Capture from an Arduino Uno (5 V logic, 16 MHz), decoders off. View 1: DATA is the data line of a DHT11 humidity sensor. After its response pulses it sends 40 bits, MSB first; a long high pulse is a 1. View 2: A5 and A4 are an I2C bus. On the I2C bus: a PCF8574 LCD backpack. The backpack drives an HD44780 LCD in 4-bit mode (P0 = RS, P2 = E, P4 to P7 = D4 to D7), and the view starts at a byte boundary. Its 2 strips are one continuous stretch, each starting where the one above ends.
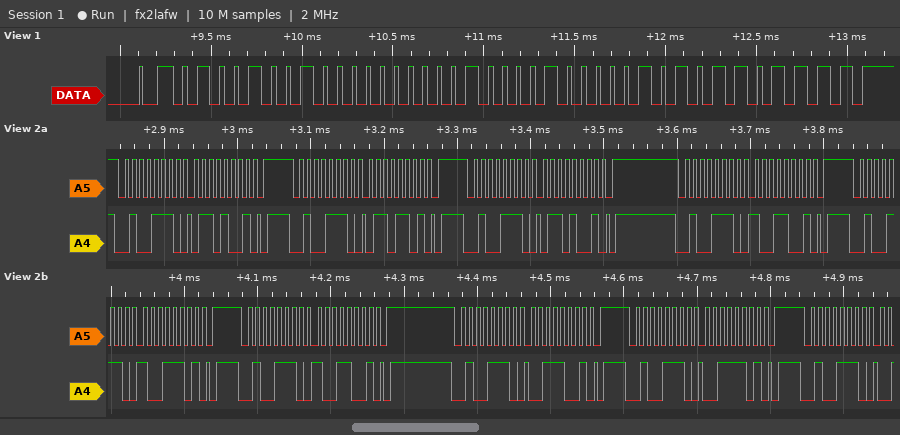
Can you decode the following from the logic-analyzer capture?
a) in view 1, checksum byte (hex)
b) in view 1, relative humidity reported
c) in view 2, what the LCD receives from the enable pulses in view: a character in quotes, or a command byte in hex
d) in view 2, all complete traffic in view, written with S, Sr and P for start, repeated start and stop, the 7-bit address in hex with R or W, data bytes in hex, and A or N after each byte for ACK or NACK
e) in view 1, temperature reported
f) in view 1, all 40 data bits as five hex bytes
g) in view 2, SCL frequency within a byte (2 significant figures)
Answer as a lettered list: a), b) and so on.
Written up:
a) 0x6F
b) 73 %
c) 'i'
d) S 27W A 69 A P S 27W A 6D A P S 27W A 69 A P S 27W A 99 A P S 27W A 9D A P S 27W A 99 A P S 27W A 39 A P S 27W A 3D A P S 27W A
e) 33.5 °C
f) 49 00 21 05 6F
g) 100 kHz
